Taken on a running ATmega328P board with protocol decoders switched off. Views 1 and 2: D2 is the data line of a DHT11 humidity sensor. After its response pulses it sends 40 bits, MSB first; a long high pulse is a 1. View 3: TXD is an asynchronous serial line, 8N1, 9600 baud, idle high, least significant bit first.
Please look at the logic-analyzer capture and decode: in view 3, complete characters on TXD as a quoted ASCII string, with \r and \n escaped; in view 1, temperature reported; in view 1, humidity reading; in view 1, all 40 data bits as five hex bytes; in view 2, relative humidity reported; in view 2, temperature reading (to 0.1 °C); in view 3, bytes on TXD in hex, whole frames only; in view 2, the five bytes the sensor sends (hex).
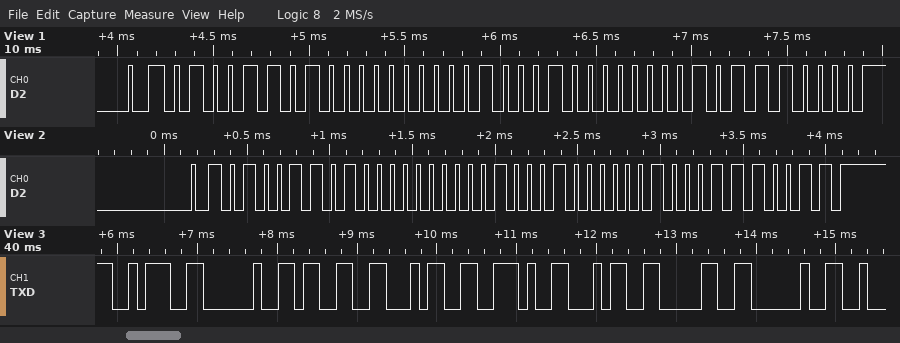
": 34.40 "
34.1 °C
77 %
4D 00 22 01 70
77 %
34.4 °C
3A 20 33 34 2E 34 30 20
4D 00 22 04 73
